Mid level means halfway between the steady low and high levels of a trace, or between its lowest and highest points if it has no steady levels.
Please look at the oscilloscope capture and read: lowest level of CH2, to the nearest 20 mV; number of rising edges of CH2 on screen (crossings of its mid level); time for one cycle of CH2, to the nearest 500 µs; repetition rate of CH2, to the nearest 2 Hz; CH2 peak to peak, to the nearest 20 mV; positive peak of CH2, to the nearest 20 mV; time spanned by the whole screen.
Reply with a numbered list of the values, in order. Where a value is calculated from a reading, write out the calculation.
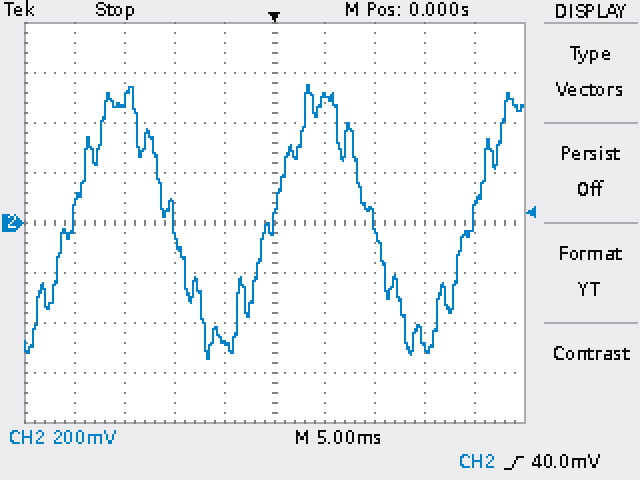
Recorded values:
1. -540 mV
2. 3
3. 20.0 ms
4. 1 / 20.0 ms ≈ 50 Hz
5. 560 mV − (-540 mV) = 1.10 V
6. 560 mV
7. 50 ms
